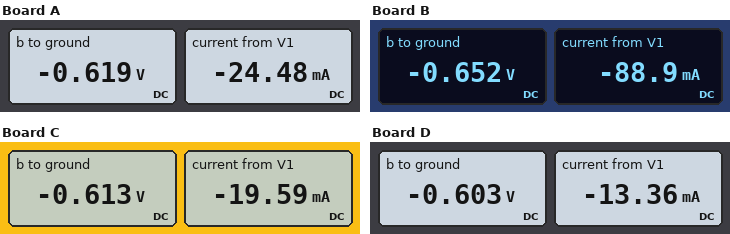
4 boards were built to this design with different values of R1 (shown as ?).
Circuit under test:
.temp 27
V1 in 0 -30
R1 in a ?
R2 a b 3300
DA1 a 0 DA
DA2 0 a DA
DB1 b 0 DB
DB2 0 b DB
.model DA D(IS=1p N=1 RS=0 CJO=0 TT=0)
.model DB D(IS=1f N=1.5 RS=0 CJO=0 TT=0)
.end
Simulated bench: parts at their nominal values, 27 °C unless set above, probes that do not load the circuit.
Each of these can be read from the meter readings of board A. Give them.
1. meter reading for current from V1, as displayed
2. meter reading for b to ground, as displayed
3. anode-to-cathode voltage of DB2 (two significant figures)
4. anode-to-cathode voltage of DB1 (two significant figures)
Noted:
-24.48 mA
-0.619 V
620 mV
-620 mV
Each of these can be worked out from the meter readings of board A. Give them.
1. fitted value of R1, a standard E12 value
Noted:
1.2 kΩ
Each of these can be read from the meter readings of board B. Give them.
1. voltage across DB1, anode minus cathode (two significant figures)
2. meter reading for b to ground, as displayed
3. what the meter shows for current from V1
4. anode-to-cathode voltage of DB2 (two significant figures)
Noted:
-650 mV
-0.652 V
-88.9 mA
650 mV
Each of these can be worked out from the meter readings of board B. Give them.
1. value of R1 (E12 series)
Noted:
330 Ω
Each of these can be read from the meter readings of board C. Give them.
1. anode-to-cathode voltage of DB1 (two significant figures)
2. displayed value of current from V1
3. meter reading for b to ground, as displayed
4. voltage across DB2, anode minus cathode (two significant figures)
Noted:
-610 mV
-19.59 mA
-0.613 V
610 mV
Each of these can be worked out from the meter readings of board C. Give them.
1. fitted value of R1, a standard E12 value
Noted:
1.5 kΩ
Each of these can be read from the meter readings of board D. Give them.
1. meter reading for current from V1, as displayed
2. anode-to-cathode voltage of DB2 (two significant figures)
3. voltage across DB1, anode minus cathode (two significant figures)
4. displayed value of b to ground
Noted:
-13.36 mA
600 mV
-600 mV
-0.603 V
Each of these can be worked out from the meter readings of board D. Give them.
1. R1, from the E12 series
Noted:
2.2 kΩ
